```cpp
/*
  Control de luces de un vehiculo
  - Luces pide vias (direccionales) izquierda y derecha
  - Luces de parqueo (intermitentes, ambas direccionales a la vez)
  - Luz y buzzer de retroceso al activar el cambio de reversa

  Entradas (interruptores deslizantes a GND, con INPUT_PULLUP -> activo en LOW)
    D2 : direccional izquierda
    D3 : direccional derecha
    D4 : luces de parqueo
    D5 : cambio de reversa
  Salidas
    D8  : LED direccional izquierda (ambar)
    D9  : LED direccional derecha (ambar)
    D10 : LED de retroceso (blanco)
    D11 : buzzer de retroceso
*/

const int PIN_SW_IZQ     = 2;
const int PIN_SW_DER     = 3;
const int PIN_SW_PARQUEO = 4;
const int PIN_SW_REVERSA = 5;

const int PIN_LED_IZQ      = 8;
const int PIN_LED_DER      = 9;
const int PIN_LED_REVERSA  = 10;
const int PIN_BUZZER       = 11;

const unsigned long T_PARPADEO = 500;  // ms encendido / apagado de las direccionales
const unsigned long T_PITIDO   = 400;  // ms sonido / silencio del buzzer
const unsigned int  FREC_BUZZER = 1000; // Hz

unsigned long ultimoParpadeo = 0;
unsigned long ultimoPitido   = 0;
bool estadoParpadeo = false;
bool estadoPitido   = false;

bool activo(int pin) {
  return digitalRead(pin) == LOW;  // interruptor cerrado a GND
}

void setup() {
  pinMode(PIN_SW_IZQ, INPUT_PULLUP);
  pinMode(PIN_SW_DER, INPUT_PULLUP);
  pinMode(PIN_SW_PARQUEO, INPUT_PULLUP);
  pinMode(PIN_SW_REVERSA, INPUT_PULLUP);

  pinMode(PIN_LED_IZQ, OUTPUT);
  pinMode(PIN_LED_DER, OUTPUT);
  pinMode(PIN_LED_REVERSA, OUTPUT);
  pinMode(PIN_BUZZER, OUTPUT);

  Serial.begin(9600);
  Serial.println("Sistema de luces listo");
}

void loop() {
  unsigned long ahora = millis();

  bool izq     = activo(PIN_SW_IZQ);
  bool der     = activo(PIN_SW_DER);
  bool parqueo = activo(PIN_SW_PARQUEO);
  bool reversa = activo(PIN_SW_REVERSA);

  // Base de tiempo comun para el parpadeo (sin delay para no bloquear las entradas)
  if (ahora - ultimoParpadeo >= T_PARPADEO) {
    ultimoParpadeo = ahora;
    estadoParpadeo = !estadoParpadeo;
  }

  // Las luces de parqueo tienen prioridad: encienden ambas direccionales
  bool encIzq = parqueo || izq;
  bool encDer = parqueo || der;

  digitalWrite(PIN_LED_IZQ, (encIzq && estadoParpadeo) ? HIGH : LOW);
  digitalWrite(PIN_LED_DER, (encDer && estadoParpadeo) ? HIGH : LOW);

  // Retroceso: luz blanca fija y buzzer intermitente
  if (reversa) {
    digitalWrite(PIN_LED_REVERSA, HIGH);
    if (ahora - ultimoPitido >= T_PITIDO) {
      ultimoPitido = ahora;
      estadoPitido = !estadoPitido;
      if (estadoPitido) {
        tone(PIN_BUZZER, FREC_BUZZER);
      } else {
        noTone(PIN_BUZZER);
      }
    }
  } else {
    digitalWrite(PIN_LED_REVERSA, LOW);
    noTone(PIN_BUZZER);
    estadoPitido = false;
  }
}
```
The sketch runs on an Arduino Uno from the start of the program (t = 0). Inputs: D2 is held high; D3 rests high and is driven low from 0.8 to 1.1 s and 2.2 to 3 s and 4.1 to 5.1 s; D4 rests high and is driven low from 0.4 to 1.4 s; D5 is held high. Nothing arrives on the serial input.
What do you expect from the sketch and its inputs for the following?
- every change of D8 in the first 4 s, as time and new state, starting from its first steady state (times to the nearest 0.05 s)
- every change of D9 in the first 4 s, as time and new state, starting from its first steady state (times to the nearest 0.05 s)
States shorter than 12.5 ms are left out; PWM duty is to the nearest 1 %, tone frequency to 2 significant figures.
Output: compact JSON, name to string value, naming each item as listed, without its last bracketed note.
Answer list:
{"every change of D8 in the first 4 s, as time and new state, starting from its first steady state": "0 s low; 0.5 s high; 1 s low", "every change of D9 in the first 4 s, as time and new state, starting from its first steady state": "0 s low; 0.5 s high; 1 s low; 2.5 s high; 3 s low"}
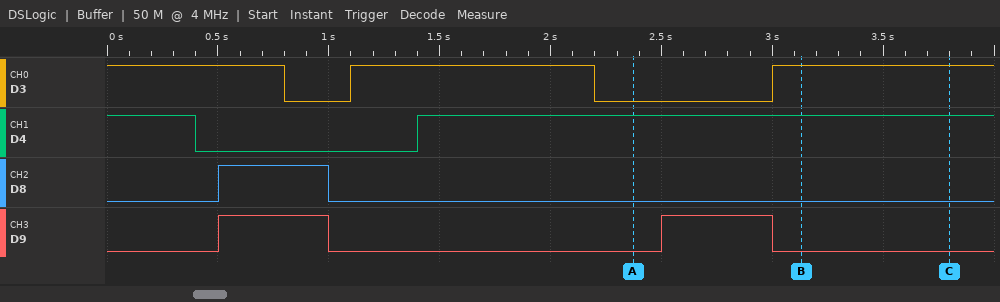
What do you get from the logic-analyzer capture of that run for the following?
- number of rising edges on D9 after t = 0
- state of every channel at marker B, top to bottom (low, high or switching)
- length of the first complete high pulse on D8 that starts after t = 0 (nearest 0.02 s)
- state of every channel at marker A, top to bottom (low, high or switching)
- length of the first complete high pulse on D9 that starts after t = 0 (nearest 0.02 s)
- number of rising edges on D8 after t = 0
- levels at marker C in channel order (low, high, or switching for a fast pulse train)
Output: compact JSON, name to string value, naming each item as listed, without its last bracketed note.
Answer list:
{"number of rising edges on D9 after t = 0": "2", "state of every channel at marker B, top to bottom": "D3 high, D4 high, D8 low, D9 low", "length of the first complete high pulse on D8 that starts after t = 0": "0.50 s", "state of every channel at marker A, top to bottom": "D3 low, D4 high, D8 low, D9 low", "length of the first complete high pulse on D9 that starts after t = 0": "0.50 s", "number of rising edges on D8 after t = 0": "1", "levels at marker C in channel order": "D3 high, D4 high, D8 low, D9 low"}
